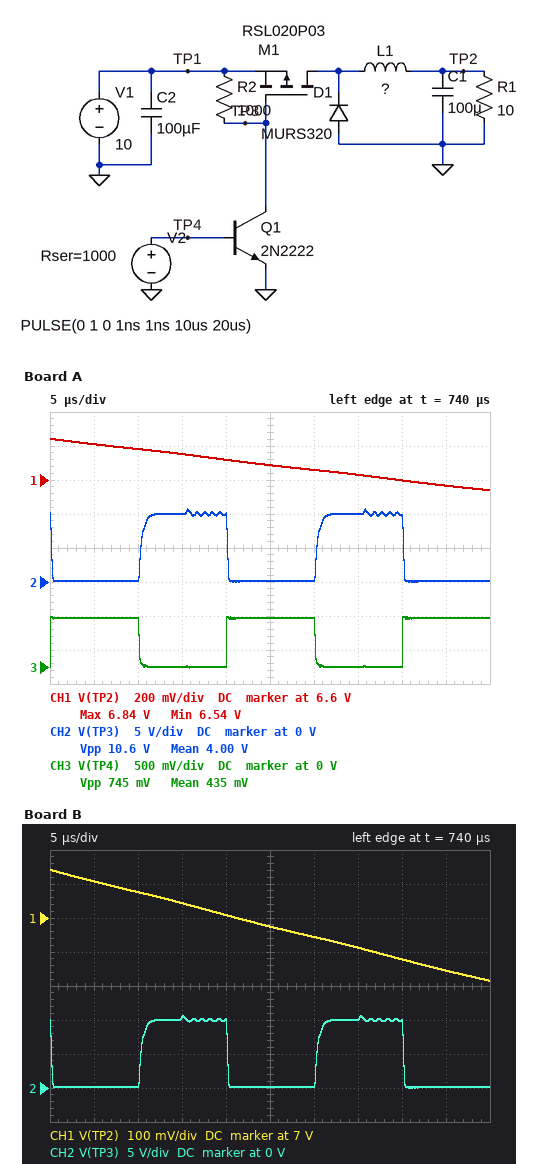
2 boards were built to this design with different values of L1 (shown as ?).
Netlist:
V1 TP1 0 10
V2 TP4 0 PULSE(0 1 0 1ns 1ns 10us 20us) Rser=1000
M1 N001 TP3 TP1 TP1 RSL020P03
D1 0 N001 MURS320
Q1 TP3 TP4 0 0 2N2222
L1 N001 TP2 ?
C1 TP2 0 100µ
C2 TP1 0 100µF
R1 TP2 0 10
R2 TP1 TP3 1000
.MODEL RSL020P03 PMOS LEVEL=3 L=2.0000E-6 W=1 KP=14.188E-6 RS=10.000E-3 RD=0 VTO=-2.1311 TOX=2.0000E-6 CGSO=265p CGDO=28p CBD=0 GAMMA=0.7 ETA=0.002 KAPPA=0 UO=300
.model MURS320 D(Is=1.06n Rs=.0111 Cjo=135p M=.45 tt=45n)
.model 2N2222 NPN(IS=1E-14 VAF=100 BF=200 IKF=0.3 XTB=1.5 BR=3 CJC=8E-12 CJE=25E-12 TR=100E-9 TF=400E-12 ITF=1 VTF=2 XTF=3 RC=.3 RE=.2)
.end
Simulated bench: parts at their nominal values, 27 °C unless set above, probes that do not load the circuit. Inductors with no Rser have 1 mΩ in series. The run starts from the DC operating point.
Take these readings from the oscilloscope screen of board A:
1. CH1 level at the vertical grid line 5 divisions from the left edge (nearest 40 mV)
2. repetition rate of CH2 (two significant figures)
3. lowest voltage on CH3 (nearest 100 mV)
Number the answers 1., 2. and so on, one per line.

1. 6.68 V
2. 50 kHz
3. 0 V
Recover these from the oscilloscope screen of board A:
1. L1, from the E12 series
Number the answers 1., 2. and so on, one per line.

1. 220 µH
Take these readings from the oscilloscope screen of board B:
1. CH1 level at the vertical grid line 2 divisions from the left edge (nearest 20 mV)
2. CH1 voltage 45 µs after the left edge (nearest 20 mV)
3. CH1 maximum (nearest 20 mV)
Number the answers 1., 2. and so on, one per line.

1. 7.08 V
2. 6.84 V
3. 7.14 V
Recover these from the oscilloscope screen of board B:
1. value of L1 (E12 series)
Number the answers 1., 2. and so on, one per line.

1. 270 µH
